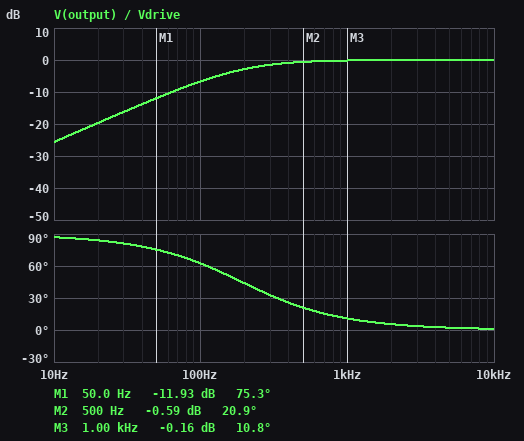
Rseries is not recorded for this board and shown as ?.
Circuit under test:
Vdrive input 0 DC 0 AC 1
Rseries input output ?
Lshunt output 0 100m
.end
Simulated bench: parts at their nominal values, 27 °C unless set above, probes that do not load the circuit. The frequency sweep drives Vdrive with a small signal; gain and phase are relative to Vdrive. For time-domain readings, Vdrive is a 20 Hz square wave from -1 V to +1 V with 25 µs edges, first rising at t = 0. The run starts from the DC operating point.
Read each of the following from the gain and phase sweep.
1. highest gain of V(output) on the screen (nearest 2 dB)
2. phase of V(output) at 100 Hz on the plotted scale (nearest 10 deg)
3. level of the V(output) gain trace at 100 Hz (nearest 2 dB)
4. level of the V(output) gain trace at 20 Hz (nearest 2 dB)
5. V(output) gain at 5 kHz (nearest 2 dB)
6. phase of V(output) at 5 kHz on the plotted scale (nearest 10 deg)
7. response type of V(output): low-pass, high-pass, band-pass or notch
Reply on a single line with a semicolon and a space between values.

0 dB; 60 deg; -6 dB; -20 dB; 0 dB; 0 deg; high-pass
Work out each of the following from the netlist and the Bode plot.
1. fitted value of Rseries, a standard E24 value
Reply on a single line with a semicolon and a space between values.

120 Ω
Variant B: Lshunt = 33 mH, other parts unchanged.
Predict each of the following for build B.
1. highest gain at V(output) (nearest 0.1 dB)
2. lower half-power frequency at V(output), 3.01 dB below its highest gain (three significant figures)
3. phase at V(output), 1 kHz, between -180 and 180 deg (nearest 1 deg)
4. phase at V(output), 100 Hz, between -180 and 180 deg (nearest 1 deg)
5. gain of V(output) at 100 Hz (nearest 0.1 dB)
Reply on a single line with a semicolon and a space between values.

0 dB; 579 Hz; 30 deg; 80 deg; -15.4 dB
